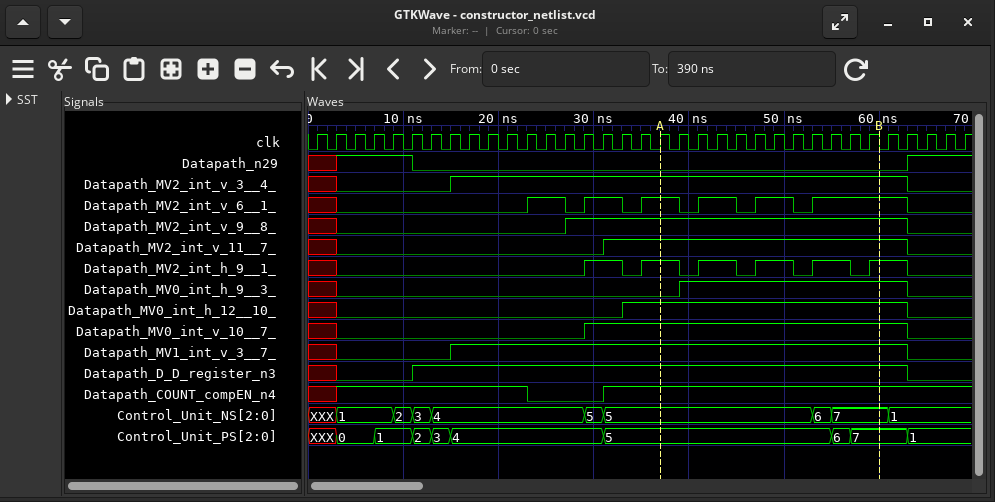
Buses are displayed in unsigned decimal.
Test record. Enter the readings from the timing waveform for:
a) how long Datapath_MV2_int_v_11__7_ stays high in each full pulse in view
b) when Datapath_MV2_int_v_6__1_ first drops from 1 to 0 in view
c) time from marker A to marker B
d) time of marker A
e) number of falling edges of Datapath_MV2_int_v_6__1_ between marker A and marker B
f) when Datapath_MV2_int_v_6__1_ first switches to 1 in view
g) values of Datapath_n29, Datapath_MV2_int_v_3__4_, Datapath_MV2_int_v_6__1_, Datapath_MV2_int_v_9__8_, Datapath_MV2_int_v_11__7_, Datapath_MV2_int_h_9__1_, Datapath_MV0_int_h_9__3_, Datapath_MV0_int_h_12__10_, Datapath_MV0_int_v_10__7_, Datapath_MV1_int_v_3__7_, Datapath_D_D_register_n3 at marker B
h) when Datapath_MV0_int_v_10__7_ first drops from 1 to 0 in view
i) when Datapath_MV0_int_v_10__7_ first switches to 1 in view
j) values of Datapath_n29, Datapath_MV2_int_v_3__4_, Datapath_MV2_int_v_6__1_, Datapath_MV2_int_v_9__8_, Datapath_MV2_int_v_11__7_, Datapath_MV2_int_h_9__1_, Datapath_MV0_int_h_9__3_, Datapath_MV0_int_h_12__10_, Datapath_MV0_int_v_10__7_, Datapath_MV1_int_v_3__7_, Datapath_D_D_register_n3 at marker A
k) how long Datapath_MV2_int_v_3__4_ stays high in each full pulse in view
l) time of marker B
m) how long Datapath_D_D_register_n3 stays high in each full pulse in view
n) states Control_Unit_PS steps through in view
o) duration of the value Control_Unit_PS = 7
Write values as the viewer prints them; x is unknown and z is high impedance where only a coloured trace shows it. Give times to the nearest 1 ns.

32 ns
27 ns
23 ns
37 ns
3
23 ns
Datapath_n29=0, Datapath_MV2_int_v_3__4_=1, Datapath_MV2_int_v_6__1_=1, Datapath_MV2_int_v_9__8_=1, Datapath_MV2_int_v_11__7_=1, Datapath_MV2_int_h_9__1_=1, Datapath_MV0_int_h_9__3_=1, Datapath_MV0_int_h_12__10_=1, Datapath_MV0_int_v_10__7_=1, Datapath_MV1_int_v_3__7_=1, Datapath_D_D_register_n3=1
63 ns
29 ns
Datapath_n29=0, Datapath_MV2_int_v_3__4_=1, Datapath_MV2_int_v_6__1_=1, Datapath_MV2_int_v_9__8_=1, Datapath_MV2_int_v_11__7_=1, Datapath_MV2_int_h_9__1_=1, Datapath_MV0_int_h_9__3_=0, Datapath_MV0_int_h_12__10_=1, Datapath_MV0_int_v_10__7_=1, Datapath_MV1_int_v_3__7_=1, Datapath_D_D_register_n3=1
48 ns
60 ns
52 ns
XXX, 0, 1, 2, 3, 4, 5, 6, 7, 1
6 ns
